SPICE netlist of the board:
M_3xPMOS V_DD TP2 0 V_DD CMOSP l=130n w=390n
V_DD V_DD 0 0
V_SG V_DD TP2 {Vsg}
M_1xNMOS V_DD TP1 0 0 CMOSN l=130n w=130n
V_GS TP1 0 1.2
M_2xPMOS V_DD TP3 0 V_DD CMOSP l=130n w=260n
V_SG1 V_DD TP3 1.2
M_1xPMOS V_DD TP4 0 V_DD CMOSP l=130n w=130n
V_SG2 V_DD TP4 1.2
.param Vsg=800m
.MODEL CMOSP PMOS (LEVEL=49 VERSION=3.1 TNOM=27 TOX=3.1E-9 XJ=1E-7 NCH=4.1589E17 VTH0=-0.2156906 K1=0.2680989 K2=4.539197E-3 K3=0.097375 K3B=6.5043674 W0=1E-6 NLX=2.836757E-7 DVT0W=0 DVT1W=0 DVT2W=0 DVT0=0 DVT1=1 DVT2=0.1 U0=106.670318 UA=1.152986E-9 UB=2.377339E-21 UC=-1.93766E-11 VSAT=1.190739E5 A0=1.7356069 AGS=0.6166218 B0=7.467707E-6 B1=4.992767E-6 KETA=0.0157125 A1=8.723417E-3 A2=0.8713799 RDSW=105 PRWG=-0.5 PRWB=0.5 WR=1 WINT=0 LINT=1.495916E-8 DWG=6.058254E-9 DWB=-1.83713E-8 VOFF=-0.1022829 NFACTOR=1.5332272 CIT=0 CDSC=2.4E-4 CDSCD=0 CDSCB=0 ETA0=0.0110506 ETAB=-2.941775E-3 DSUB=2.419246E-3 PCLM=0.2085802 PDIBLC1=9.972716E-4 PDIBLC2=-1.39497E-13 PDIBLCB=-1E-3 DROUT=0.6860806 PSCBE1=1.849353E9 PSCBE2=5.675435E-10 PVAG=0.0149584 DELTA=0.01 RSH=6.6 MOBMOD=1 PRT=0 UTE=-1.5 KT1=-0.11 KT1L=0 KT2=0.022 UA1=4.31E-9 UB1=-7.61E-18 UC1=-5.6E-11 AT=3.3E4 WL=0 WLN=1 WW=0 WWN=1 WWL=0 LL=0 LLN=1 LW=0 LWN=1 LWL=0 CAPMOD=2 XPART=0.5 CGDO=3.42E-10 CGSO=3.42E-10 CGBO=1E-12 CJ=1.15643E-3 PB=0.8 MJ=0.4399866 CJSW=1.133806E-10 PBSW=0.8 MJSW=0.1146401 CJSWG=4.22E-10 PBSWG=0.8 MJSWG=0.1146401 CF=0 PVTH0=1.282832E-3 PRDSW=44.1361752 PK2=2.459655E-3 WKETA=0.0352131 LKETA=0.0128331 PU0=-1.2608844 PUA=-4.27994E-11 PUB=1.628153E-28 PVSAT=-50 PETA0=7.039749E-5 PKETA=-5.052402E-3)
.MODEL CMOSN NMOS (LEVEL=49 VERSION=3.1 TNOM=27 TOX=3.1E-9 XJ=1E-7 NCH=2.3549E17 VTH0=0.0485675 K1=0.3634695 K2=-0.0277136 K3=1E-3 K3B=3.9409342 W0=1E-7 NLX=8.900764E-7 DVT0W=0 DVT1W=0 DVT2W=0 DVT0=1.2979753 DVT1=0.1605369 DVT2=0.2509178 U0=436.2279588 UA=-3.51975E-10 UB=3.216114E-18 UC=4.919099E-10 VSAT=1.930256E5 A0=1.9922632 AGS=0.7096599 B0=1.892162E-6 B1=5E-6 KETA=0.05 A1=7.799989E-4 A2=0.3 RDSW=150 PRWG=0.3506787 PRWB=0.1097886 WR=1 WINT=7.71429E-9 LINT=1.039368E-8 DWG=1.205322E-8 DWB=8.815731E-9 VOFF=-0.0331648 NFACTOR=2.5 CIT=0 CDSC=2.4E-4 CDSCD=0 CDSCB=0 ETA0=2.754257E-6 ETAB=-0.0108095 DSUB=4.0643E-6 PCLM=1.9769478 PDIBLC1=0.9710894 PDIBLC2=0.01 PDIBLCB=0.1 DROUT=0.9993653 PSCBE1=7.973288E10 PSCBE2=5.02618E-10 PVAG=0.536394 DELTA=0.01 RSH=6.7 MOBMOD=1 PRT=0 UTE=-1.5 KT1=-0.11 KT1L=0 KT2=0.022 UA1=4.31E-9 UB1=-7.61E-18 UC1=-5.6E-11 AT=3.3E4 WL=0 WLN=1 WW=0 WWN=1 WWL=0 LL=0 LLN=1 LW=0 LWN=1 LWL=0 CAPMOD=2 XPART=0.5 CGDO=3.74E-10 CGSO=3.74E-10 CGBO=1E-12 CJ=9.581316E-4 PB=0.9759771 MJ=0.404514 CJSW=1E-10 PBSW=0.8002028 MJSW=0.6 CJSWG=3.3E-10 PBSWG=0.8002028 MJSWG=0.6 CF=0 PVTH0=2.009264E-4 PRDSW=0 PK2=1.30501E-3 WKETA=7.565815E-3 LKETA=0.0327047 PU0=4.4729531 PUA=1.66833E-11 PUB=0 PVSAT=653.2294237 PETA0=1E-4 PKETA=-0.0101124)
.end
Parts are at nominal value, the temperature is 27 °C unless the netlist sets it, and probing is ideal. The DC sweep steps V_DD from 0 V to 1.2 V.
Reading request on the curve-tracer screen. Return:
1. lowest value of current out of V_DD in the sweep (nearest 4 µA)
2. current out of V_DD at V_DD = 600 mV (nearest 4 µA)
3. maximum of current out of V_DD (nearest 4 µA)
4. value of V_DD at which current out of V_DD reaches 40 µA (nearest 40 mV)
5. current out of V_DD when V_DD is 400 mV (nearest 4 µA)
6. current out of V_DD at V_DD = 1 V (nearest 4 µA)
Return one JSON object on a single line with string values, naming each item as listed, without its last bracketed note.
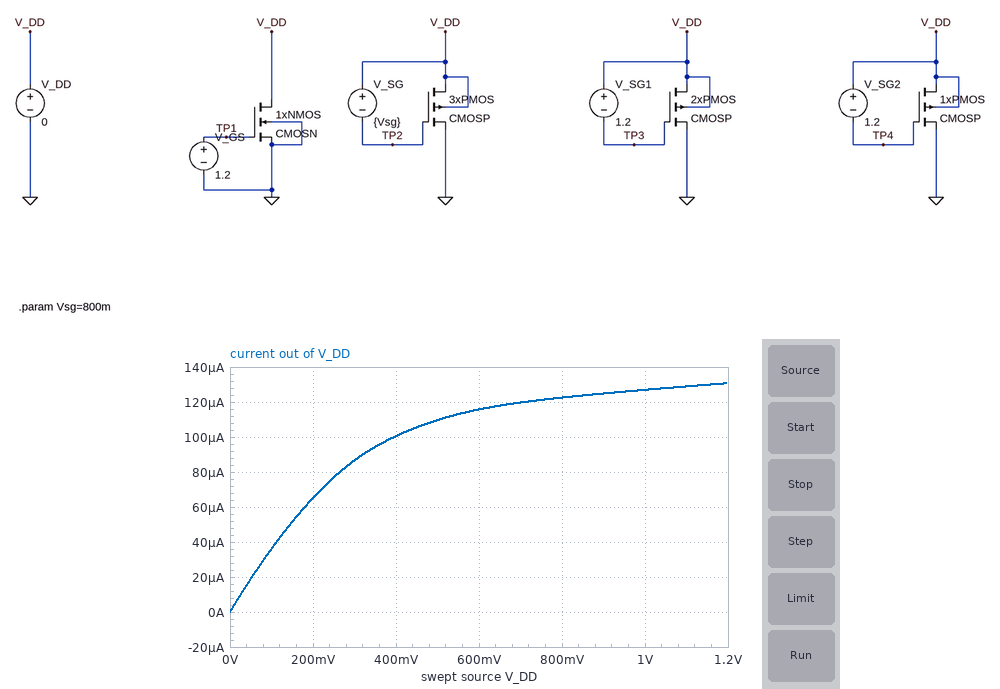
{"lowest value of current out of V_DD in the sweep": "0 A", "current out of V_DD at V_DD = 600 mV": "116 µA", "maximum of current out of V_DD": "132 µA", "value of V_DD at which current out of V_DD reaches 40 µA": "120 mV", "current out of V_DD when V_DD is 400 mV": "100 µA", "current out of V_DD at V_DD = 1 V": "128 µA"}
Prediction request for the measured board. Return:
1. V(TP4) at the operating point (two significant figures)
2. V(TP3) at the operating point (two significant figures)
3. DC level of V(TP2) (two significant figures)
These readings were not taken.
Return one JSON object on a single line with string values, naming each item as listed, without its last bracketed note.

{"V(TP4) at the operating point": "-1.2 V", "V(TP3) at the operating point": "-1.2 V", "DC level of V(TP2)": "-800 mV"}
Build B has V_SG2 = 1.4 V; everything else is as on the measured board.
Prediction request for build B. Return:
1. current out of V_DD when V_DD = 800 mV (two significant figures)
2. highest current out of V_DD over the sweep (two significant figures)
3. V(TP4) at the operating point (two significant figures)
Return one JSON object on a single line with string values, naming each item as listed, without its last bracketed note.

{"current out of V_DD when V_DD = 800 mV": "130 µA", "highest current out of V_DD over the sweep": "140 µA", "V(TP4) at the operating point": "-1.4 V"}
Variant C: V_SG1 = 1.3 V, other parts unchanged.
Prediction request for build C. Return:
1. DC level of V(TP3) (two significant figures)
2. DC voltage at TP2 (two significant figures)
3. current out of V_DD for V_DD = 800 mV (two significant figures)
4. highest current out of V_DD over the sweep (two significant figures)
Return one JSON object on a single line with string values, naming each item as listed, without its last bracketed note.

{"DC level of V(TP3)": "-1.3 V", "DC voltage at TP2": "-800 mV", "current out of V_DD for V_DD = 800 mV": "130 µA", "highest current out of V_DD over the sweep": "140 µA"}
